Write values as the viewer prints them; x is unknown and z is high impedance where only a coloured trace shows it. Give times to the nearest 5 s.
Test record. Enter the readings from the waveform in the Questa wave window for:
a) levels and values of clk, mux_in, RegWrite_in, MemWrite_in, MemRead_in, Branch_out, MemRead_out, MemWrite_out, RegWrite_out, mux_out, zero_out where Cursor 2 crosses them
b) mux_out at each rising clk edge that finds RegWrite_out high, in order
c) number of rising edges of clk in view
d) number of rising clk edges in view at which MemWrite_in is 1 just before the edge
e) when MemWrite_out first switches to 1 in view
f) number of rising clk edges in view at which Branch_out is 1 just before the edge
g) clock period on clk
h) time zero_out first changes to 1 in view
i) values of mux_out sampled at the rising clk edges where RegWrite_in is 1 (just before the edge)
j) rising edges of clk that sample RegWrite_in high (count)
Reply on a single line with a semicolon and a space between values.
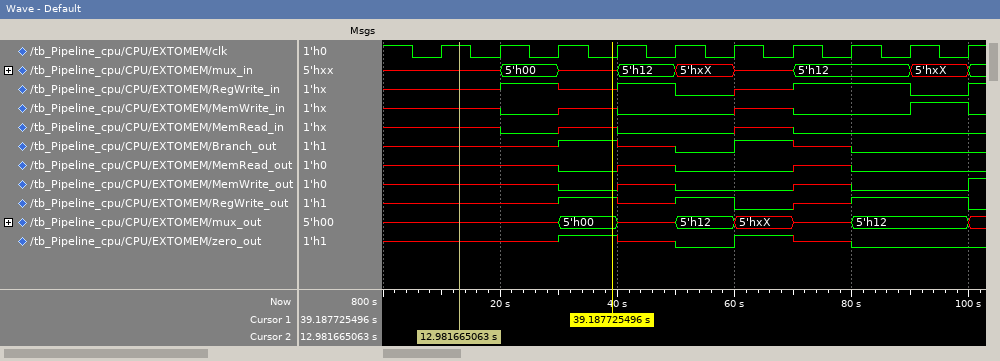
clk=1, mux_in=x, RegWrite_in=x, MemWrite_in=x, MemRead_in=x, Branch_out=x, MemRead_out=x, MemWrite_out=x, RegWrite_out=x, mux_out=x, zero_out=x; 5'h00, 5'h12, 5'h12, 5'h12; 10; 1; 100 s; 2; 10 s; 30 s; x, x, x, 5'h12; 4
